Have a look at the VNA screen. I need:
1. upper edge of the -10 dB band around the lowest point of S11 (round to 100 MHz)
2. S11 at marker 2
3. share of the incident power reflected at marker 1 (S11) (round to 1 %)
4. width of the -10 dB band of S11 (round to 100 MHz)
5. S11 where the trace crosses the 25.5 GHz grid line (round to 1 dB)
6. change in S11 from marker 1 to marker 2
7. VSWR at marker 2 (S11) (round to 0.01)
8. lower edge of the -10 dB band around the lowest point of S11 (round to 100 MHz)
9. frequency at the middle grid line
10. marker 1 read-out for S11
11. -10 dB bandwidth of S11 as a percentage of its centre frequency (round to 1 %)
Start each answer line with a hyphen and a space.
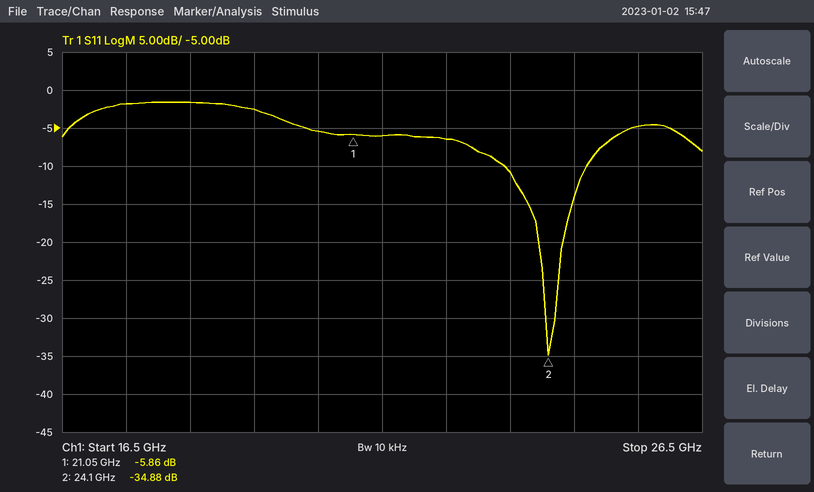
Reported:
- 24.7 GHz
- -34.88 dB
- 26 %
- 1.3 GHz
- -5 dB
- -29.02 dB
- 1.04
- 23.4 GHz
- 21.5 GHz
- -5.86 dB
- 5 %
